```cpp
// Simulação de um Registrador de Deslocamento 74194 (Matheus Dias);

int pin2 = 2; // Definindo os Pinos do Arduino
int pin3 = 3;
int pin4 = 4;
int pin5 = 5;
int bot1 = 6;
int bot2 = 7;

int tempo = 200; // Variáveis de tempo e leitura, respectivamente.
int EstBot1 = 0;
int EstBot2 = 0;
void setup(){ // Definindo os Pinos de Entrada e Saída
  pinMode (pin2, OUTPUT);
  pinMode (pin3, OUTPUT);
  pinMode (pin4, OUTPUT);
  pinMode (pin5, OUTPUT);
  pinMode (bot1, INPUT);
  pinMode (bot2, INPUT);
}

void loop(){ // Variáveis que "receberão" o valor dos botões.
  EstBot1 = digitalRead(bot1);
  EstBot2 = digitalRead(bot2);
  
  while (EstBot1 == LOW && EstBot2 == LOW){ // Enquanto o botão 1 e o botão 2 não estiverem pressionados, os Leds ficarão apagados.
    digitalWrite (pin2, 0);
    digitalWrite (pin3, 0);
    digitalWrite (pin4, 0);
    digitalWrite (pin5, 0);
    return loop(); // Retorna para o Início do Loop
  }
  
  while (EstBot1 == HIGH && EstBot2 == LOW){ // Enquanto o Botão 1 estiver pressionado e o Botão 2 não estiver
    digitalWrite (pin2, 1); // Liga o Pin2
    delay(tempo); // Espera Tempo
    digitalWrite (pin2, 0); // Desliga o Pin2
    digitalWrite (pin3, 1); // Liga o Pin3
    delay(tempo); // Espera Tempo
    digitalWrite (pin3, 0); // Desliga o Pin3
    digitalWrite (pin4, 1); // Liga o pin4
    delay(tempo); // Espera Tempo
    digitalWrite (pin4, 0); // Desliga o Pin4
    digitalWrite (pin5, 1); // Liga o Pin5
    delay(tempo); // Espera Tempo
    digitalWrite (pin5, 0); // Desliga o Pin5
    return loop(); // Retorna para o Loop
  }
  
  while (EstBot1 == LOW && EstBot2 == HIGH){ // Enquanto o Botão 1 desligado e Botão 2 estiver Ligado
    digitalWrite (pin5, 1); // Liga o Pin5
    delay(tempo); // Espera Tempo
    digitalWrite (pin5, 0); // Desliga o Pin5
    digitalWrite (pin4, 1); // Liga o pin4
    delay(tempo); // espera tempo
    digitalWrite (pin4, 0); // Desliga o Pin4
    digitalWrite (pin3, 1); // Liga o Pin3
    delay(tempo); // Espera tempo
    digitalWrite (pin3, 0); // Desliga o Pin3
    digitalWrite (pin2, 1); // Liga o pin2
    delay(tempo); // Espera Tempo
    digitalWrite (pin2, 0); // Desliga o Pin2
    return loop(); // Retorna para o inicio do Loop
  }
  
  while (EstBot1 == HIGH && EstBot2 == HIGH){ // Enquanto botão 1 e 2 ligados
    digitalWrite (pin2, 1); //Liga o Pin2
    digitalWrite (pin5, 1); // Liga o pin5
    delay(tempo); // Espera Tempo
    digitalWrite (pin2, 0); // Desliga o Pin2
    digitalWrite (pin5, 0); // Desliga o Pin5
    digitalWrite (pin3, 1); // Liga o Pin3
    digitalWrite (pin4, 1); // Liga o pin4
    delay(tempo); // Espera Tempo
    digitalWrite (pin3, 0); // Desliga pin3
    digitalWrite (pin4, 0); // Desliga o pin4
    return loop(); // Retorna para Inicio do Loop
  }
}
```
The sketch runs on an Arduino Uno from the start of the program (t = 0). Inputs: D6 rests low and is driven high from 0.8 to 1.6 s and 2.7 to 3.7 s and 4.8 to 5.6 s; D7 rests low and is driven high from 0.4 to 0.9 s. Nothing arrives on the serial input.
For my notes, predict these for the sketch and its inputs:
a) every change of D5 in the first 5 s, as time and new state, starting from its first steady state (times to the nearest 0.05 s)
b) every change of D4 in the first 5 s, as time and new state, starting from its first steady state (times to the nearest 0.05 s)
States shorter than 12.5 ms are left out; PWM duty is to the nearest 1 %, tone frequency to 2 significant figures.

0 s low; 0.4 s high; 0.6 s low; 1.8 s high; 2 s low; 3.3 s high; 3.5 s low; 4.1 s high; 4.3 s low
0 s low; 0.6 s high; 0.8 s low; 1.6 s high; 1.8 s low; 3.1 s high; 3.3 s low; 3.9 s high; 4.1 s low
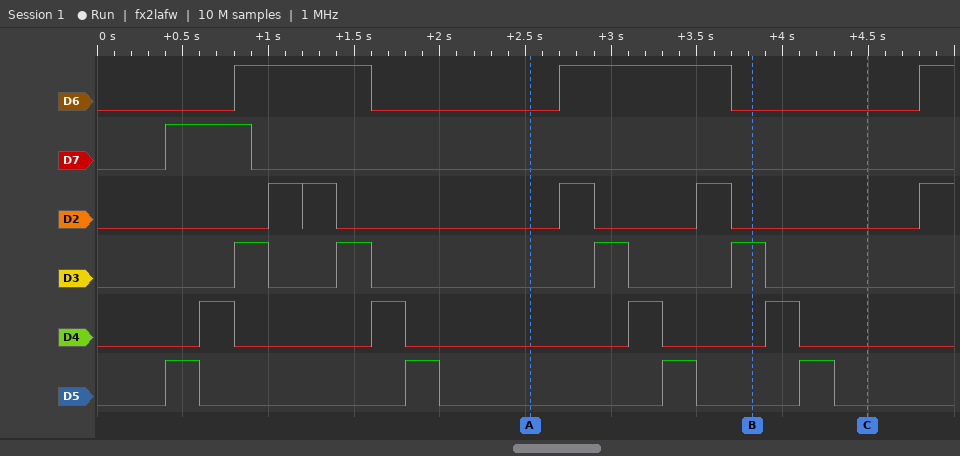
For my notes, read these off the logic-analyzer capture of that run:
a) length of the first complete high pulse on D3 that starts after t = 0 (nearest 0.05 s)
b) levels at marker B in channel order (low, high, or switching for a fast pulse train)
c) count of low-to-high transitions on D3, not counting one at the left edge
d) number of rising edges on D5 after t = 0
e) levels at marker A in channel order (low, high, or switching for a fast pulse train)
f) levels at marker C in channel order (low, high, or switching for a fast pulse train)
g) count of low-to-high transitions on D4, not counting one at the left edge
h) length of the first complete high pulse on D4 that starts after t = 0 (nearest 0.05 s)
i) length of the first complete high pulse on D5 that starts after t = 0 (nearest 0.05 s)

0.20 s
D6 low, D7 low, D2 low, D3 high, D4 low, D5 low
4
4
D6 low, D7 low, D2 low, D3 low, D4 low, D5 low
D6 low, D7 low, D2 low, D3 low, D4 low, D5 low
4
0.20 s
0.20 s
